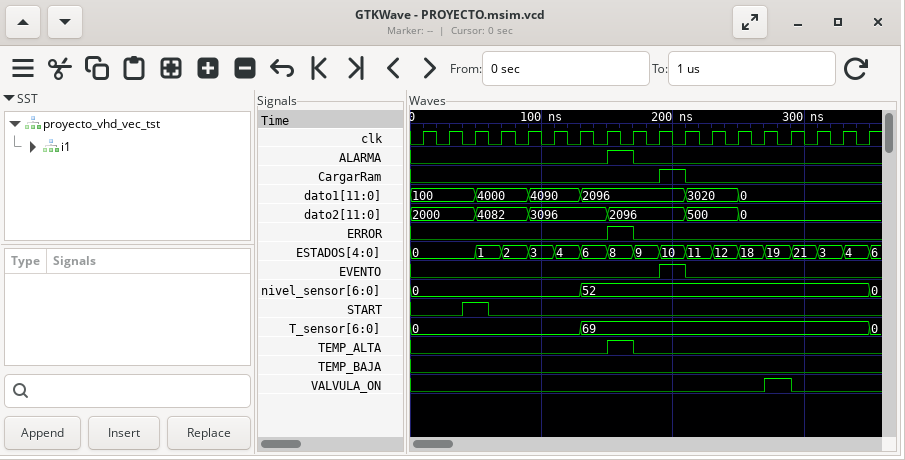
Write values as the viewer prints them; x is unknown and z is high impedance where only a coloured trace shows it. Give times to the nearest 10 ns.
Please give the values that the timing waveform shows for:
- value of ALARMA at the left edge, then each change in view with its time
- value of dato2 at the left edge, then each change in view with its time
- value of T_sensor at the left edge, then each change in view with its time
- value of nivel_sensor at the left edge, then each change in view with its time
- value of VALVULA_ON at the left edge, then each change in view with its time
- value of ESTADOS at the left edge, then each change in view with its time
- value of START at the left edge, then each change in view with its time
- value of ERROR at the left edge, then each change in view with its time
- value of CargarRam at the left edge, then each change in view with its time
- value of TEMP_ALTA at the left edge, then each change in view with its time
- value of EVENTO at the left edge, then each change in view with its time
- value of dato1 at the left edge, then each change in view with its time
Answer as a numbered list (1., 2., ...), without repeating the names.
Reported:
1. 0, 1 at 150 ns, 0 at 170 ns
2. 2000, 4082 at 50 ns, 3096 at 90 ns, 2096 at 150 ns, 500 at 210 ns, 0 at 250 ns
3. 0, 69 at 130 ns, 0 at 350 ns
4. 0, 52 at 130 ns, 0 at 350 ns
5. 0, 1 at 270 ns, 0 at 290 ns
6. 0, 1 at 50 ns, 2 at 70 ns, 3 at 90 ns, 4 at 110 ns, 6 at 130 ns, 8 at 150 ns, 9 at 170 ns, 10 at 190 ns, 11 at 210 ns, 12 at 230 ns, 18 at 250 ns, 19 at 270 ns, 21 at 290 ns, 3 at 310 ns, 4 at 330 ns, 6 at 350 ns
7. 0, 1 at 40 ns, 0 at 60 ns
8. 0, 1 at 150 ns, 0 at 170 ns
9. 0, 1 at 190 ns, 0 at 210 ns
10. 0, 1 at 150 ns, 0 at 170 ns
11. 0, 1 at 190 ns, 0 at 210 ns
12. 100, 4000 at 50 ns, 4090 at 90 ns, 2096 at 130 ns, 3020 at 210 ns, 0 at 250 ns
